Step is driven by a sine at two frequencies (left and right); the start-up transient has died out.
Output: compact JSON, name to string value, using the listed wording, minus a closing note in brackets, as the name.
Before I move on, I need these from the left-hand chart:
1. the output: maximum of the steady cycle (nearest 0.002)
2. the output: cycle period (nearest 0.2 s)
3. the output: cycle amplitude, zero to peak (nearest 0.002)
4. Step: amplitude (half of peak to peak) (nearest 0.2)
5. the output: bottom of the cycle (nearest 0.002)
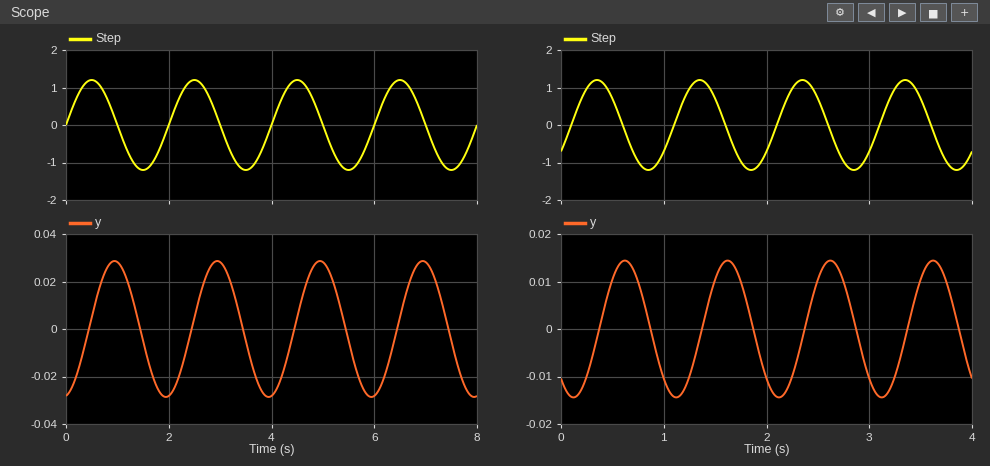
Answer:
{"the output: maximum of the steady cycle": "0.028", "the output: cycle period": "2.0 s", "the output: cycle amplitude, zero to peak": "0.028", "Step: amplitude (half of peak to peak)": "1.2", "the output: bottom of the cycle": "-0.028"}
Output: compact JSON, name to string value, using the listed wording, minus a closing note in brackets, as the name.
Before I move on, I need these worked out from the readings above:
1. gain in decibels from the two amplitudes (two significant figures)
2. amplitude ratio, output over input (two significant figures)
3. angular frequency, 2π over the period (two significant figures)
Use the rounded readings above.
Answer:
{"gain in decibels from the two amplitudes": "-33 dB", "amplitude ratio, output over input": "0.023", "angular frequency, 2π over the period": "3.1 rad/s"}
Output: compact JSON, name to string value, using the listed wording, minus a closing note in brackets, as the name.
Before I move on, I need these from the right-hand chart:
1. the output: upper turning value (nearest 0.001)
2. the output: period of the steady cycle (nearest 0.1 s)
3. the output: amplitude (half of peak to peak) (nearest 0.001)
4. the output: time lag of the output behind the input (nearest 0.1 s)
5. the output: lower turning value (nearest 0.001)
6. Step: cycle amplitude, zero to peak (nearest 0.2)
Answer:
{"the output: upper turning value": "0.014", "the output: period of the steady cycle": "1.0 s", "the output: amplitude (half of peak to peak)": "0.014", "the output: time lag of the output behind the input": "0.3 s", "the output: lower turning value": "-0.014", "Step: cycle amplitude, zero to peak": "1.2"}
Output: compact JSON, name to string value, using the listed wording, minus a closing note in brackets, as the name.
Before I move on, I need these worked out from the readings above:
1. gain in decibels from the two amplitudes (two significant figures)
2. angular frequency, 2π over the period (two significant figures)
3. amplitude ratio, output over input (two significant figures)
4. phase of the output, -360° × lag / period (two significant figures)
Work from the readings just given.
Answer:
{"gain in decibels from the two amplitudes": "-39 dB", "angular frequency, 2π over the period": "6.3 rad/s", "amplitude ratio, output over input": "0.012", "phase of the output, -360° × lag / period": "-110°"}
